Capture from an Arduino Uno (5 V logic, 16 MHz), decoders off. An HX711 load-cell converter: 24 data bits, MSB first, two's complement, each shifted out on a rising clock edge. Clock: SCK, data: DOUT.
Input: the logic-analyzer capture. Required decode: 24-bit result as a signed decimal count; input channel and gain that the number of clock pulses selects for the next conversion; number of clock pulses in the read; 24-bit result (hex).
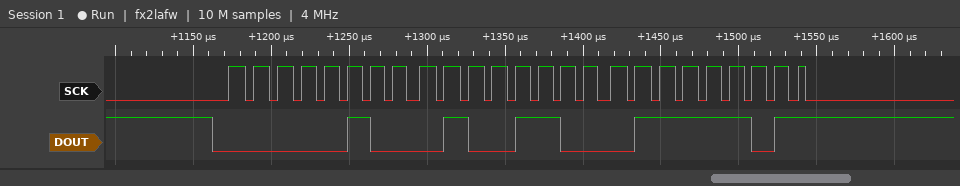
281725
channel A, gain 128
25
0x044C7D
